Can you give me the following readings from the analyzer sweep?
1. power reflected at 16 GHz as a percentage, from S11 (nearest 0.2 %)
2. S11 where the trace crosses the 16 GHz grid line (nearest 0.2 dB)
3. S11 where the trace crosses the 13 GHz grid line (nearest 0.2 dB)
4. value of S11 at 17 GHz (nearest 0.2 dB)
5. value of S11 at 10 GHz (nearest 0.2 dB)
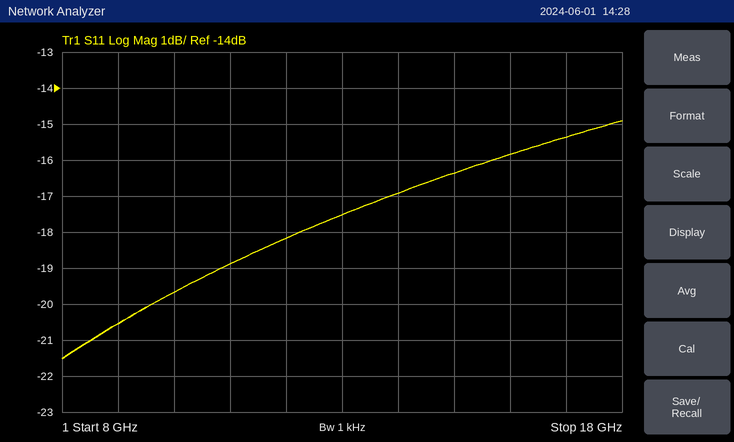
2.6 %
-15.8 dB
-17.6 dB
-15.4 dB
-19.6 dB
